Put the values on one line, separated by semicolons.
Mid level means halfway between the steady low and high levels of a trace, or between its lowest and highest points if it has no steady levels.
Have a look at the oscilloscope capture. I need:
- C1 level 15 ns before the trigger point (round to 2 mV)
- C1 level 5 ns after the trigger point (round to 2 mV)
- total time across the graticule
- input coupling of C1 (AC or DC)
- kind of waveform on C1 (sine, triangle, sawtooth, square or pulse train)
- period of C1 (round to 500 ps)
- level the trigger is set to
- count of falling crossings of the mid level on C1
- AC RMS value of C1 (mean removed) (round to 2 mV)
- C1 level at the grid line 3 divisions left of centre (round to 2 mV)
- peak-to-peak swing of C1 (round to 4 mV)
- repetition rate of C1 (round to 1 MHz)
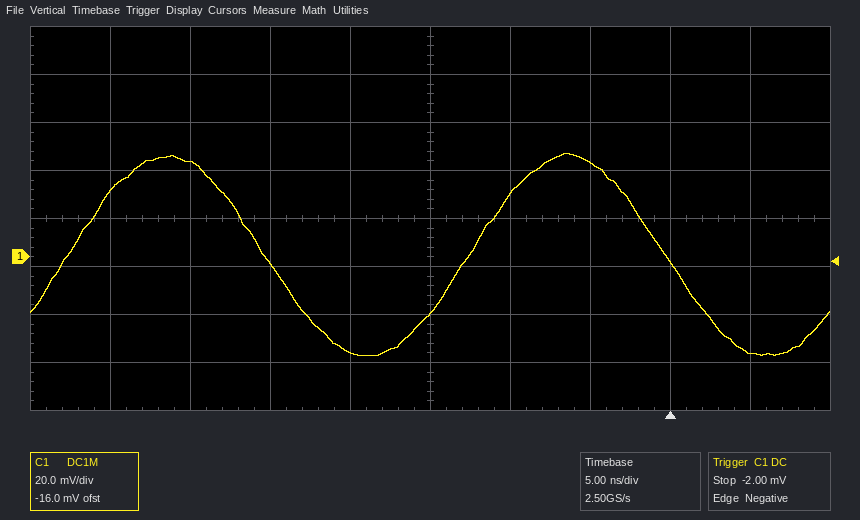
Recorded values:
-24 mV; -40 mV; 50 ns; DC; sine; 25.0 ns; -2.00 mV; 2; 30 mV; 40 mV; 84 mV; 40 MHz
